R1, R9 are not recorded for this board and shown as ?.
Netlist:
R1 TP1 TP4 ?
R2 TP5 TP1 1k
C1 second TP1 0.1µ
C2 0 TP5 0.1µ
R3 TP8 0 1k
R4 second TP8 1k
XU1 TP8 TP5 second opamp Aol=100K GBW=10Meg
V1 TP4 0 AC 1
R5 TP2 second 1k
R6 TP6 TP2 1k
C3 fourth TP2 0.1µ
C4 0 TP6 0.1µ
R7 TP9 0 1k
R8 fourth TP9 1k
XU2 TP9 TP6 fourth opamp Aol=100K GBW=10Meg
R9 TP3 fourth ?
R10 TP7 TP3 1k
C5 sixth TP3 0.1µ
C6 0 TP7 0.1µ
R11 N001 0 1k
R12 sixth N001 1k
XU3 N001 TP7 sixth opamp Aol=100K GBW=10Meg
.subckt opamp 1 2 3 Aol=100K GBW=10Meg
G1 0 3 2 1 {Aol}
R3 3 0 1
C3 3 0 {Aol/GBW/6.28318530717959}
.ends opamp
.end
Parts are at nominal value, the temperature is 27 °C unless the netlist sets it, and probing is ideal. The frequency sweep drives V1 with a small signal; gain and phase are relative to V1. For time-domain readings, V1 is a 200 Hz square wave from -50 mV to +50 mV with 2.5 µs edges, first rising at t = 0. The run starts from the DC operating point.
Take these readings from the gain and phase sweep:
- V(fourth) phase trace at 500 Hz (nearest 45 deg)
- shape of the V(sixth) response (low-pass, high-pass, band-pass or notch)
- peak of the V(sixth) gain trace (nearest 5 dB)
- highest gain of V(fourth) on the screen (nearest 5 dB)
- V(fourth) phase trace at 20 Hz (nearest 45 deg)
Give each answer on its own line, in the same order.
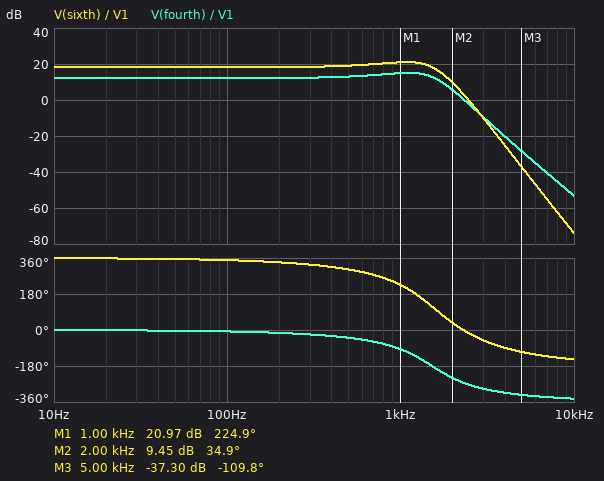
-45 deg
low-pass
20 dB
15 dB
0 deg
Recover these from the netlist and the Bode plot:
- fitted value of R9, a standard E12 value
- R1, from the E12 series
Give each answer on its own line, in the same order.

560 Ω
1.2 kΩ
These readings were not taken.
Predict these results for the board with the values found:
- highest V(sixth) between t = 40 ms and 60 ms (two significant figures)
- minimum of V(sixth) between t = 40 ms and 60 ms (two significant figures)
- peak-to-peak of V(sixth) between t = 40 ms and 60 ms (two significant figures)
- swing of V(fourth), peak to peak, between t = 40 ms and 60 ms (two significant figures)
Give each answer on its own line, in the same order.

660 mV
-660 mV
1.3 V
650 mV
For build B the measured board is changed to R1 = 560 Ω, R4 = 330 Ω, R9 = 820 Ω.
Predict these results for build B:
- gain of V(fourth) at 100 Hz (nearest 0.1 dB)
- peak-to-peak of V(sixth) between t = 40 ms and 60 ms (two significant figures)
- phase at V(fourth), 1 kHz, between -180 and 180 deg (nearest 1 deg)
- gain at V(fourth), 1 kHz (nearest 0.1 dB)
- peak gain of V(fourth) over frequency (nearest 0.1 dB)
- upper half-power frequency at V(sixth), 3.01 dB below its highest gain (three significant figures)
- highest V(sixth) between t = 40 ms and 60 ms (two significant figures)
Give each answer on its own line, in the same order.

8.5 dB
710 mV
-94 deg
8.4 dB
8.6 dB
1.51 kHz
350 mV
